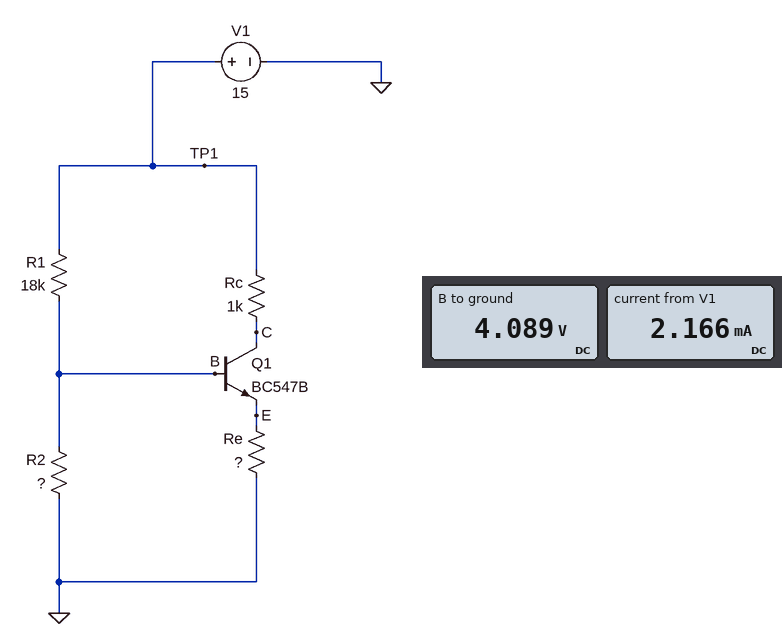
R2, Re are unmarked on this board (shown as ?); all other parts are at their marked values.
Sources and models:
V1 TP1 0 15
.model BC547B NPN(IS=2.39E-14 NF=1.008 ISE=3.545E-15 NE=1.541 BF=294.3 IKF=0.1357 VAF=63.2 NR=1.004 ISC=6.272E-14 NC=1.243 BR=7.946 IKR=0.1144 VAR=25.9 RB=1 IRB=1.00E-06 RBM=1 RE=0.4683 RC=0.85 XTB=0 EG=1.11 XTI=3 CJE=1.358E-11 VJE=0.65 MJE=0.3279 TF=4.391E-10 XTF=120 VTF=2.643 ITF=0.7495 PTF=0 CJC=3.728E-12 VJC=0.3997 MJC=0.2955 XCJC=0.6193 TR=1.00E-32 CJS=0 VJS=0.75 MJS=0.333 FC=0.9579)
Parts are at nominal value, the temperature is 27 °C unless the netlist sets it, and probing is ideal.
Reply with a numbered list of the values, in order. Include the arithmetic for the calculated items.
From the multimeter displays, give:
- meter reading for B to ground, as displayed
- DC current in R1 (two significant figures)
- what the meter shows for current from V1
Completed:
1. 4.089 V
2. (15 V - 4.089 V) / 18 kΩ = 610 µA
3. 2.166 mA
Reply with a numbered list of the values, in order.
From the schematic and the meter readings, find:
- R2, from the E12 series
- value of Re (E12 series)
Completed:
1. 6.8 kΩ
2. 2.2 kΩ
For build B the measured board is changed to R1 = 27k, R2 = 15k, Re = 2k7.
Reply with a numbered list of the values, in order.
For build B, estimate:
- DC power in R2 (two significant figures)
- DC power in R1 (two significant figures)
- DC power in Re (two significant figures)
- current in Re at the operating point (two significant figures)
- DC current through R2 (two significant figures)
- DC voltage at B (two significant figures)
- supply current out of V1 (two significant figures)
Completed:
1. 1.9 mW
2. 3.5 mW
3. 8.0 mW
4. 1.7 mA
5. 350 µA
6. 5.3 V
7. 2.1 mA
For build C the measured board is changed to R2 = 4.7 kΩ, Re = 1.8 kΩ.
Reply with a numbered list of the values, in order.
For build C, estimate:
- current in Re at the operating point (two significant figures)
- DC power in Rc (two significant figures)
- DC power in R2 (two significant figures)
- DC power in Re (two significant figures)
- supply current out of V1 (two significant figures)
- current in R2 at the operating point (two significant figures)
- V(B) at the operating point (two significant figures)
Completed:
1. 1.4 mA
2. 1.8 mW
3. 2.0 mW
4. 3.3 mW
5. 2.0 mA
6. 660 µA
7. 3.1 V
